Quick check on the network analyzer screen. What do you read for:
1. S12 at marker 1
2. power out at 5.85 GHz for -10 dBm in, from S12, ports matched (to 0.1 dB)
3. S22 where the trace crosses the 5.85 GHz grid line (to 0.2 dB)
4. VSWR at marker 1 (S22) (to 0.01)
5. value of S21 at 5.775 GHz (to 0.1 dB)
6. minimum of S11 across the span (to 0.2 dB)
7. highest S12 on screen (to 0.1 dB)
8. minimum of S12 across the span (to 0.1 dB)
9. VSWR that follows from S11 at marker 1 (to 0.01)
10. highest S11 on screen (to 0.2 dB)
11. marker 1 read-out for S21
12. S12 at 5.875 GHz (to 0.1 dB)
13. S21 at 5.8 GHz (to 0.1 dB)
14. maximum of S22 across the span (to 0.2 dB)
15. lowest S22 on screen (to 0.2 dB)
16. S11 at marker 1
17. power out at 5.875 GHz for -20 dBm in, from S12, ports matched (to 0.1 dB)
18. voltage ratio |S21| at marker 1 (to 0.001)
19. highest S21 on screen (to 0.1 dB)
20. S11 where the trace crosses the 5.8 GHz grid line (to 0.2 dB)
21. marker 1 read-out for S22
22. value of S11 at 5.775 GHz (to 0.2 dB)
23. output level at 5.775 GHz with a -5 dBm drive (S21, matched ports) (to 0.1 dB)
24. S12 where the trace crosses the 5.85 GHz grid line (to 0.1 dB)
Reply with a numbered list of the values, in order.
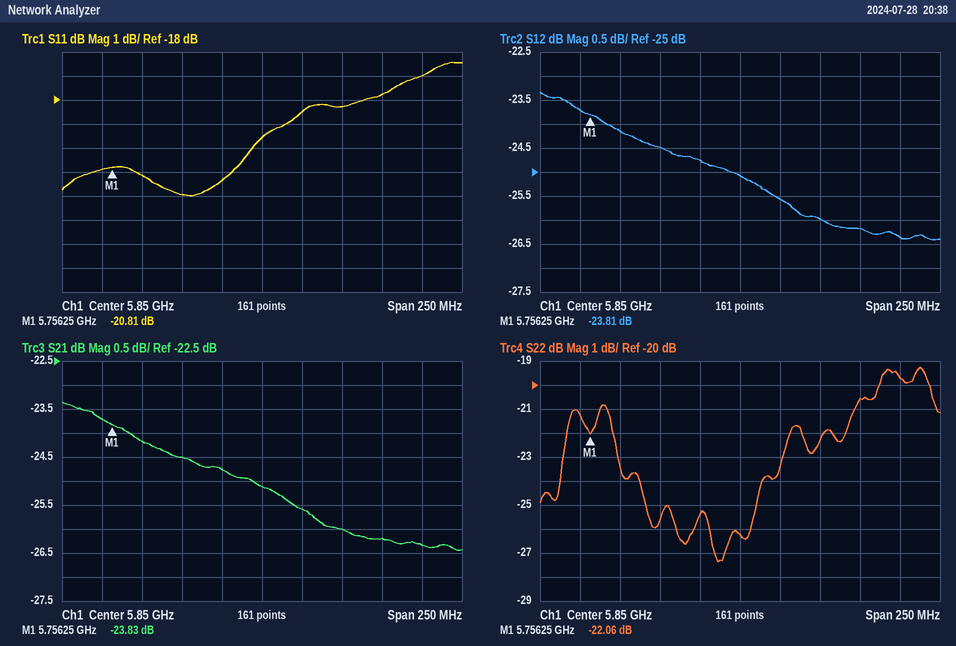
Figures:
1. -23.81 dB
2. -35.1 dBm
3. -26.2 dB
4. 1.17
5. -24.2 dB
6. -22.0 dB
7. -23.3 dB
8. -26.4 dB
9. 1.20
10. -16.4 dB
11. -23.83 dB
12. -25.6 dB
13. -24.5 dB
14. -19.2 dB
15. -27.4 dB
16. -20.81 dB
17. -45.6 dBm
18. 0.064
19. -23.4 dB
20. -22.0 dB
21. -22.06 dB
22. -21.2 dB
23. -29.2 dBm
24. -25.1 dB
